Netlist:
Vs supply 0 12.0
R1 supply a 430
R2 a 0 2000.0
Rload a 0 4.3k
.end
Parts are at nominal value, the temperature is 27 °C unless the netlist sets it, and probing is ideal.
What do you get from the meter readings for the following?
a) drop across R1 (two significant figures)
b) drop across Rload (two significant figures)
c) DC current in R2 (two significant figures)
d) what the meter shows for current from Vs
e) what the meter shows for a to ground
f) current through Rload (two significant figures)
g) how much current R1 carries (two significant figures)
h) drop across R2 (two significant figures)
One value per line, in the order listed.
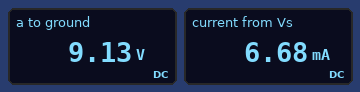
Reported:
2.9 V
9.1 V
4.6 mA
6.68 mA
9.13 V
2.1 mA
6.7 mA
9.1 V
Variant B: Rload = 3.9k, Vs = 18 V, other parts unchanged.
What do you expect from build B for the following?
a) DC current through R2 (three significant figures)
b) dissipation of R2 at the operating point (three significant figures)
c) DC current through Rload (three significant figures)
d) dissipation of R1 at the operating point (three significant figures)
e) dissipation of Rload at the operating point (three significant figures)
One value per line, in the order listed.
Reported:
6.79 mA
92.2 mW
3.48 mA
45.4 mW
47.3 mW
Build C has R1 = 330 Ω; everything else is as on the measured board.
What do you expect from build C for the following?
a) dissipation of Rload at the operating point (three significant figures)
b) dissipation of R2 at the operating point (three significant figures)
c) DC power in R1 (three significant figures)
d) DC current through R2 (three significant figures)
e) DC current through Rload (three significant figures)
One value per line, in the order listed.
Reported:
21.7 mW
46.7 mW
16.5 mW
4.83 mA
2.25 mA
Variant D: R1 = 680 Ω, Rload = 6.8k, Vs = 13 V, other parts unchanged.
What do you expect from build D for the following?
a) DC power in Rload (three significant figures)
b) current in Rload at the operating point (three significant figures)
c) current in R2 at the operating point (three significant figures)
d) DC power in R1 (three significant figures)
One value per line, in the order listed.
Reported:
12.0 mW
1.33 mA
4.51 mA
23.2 mW
